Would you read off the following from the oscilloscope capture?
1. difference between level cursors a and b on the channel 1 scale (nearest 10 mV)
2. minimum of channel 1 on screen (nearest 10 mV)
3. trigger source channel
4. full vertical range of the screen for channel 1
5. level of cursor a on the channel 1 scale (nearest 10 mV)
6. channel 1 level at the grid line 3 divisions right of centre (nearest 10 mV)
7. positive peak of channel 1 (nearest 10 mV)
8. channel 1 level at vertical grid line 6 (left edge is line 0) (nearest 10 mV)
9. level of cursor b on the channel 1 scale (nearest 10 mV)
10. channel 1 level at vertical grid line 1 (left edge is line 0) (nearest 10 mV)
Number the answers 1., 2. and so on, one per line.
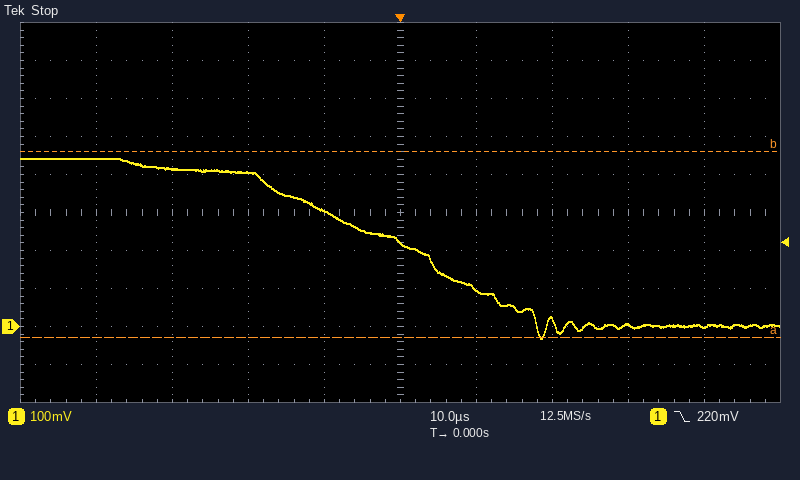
1. 490 mV
2. -30 mV
3. channel 1
4. 1 V
5. -30 mV
6. 0 mV
7. 440 mV
8. 100 mV
9. 460 mV
10. 440 mV
